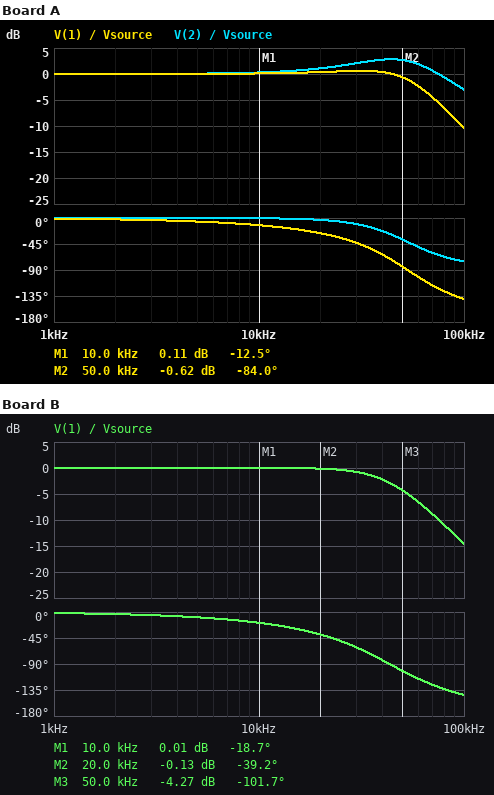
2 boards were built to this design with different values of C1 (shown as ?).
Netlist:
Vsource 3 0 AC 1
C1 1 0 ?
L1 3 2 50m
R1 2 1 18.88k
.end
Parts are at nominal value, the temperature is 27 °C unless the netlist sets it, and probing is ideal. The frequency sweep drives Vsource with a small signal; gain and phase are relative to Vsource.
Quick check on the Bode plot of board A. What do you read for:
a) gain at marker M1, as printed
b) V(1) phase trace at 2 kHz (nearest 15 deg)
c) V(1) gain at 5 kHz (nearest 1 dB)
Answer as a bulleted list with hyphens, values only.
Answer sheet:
- 0.11 dB
- 0 deg
- 0 dB
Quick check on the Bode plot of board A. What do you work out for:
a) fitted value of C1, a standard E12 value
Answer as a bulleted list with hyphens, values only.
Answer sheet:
- 180 pF
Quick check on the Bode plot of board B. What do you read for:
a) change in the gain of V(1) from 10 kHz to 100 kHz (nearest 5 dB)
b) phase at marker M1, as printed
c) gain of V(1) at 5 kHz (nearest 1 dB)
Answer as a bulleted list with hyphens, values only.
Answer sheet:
- -15 dB
- -18.7 deg
- 0 dB
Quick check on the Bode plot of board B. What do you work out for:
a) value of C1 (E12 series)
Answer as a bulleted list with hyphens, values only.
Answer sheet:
- 270 pF
